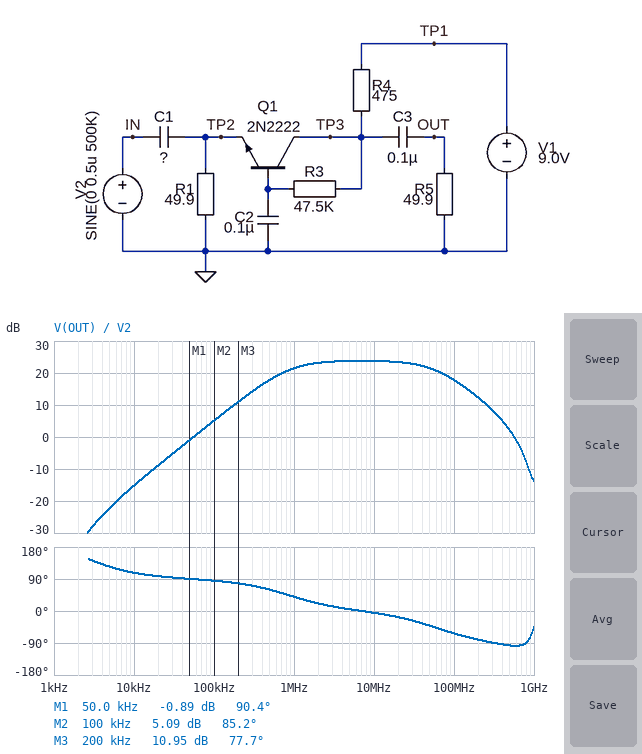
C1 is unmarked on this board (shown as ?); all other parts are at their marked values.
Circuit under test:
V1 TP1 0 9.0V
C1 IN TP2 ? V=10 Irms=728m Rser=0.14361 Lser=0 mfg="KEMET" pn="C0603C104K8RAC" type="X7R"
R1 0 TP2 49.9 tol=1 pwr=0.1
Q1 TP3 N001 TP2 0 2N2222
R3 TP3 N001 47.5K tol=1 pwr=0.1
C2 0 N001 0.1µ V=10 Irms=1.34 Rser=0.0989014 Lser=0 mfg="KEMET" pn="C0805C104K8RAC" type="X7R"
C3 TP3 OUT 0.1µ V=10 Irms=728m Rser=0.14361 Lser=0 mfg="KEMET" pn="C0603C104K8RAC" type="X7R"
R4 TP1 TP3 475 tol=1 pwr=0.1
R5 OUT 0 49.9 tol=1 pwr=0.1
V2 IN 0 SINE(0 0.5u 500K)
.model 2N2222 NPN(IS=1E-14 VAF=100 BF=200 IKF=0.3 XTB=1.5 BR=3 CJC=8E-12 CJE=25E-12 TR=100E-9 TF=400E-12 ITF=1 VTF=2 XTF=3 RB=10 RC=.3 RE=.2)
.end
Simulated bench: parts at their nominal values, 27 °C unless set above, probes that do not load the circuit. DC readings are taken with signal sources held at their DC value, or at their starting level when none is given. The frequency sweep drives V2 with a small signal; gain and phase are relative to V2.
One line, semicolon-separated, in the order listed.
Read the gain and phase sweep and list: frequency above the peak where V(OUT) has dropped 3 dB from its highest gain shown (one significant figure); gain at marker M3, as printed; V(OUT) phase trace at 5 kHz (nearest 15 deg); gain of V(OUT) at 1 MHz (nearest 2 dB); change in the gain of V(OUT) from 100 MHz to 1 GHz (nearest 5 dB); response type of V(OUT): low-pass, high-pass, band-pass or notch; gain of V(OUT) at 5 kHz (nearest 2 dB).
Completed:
60 MHz; 10.95 dB; 120 deg; 22 dB; -30 dB; band-pass; -22 dB
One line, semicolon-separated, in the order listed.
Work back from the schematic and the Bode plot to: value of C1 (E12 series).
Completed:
68 nF
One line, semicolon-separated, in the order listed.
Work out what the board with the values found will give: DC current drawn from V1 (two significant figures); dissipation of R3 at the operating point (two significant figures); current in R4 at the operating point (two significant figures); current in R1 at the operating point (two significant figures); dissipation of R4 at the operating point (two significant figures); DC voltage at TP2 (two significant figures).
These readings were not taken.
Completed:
11 mA; 140 µW; 11 mA; 11 mA; 56 mW; 540 mV
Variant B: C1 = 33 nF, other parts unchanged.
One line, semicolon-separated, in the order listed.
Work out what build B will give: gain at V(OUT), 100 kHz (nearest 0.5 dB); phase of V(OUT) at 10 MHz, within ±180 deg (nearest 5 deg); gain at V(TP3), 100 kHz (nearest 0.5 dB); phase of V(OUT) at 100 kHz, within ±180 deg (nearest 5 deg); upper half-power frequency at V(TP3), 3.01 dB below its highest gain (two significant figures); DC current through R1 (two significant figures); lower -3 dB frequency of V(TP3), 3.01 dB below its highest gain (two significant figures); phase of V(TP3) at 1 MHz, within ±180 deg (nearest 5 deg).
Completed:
-1.0 dB; 0 deg; -0.5 dB; 90 deg; 60 MHz; 11 mA; 1.7 MHz; 60 deg
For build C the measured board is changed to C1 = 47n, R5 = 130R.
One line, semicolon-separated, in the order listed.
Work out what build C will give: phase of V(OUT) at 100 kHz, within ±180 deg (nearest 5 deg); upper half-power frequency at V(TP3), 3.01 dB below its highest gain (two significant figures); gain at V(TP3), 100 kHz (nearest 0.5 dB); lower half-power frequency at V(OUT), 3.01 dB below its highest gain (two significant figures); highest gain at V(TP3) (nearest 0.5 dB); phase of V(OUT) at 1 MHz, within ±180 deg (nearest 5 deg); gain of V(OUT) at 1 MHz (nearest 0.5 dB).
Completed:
85 deg; 43 MHz; 9.0 dB; 1.2 MHz; 31.0 dB; 50 deg; 27.0 dB
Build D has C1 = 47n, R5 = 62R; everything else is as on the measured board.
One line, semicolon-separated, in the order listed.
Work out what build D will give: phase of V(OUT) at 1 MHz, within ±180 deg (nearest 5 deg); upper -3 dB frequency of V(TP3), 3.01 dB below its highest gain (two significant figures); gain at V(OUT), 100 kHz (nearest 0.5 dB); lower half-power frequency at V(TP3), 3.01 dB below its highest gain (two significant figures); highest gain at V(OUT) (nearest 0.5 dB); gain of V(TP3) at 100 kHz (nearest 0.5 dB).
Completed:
50 deg; 56 MHz; 3.5 dB; 1.2 MHz; 25.5 dB; 4.0 dB
